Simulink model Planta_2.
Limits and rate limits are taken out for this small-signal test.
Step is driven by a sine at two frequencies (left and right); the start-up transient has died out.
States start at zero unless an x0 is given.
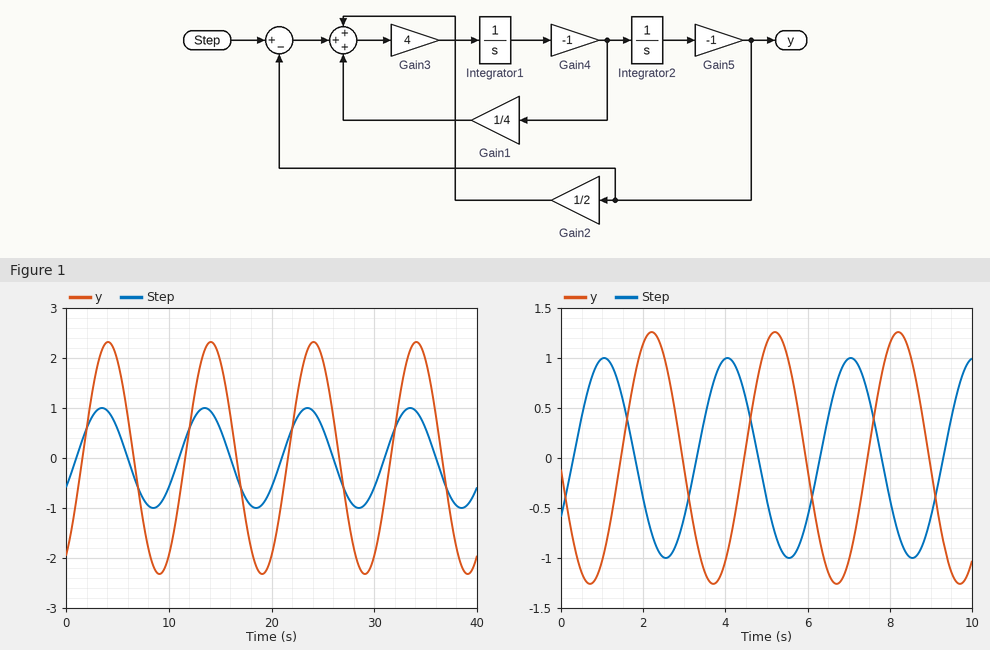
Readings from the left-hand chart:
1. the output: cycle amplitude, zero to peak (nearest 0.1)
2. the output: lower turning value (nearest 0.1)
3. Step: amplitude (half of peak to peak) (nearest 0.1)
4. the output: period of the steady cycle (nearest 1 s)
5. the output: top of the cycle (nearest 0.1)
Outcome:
2.3
-2.3
1.0
10 s
2.3
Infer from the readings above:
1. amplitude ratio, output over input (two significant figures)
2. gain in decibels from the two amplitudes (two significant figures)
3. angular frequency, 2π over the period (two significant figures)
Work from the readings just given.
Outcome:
2.3
7.2 dB
0.63 rad/s
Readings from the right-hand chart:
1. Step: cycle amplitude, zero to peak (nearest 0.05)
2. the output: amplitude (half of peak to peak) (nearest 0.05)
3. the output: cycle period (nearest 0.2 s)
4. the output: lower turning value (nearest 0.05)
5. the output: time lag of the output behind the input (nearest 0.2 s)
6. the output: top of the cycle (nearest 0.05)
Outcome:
1.00
1.25
3.0 s
-1.25
1.2 s
1.25
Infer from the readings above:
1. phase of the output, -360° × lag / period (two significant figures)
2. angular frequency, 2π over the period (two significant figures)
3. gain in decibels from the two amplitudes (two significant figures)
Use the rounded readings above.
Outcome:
-140°
2.1 rad/s
1.9 dB
